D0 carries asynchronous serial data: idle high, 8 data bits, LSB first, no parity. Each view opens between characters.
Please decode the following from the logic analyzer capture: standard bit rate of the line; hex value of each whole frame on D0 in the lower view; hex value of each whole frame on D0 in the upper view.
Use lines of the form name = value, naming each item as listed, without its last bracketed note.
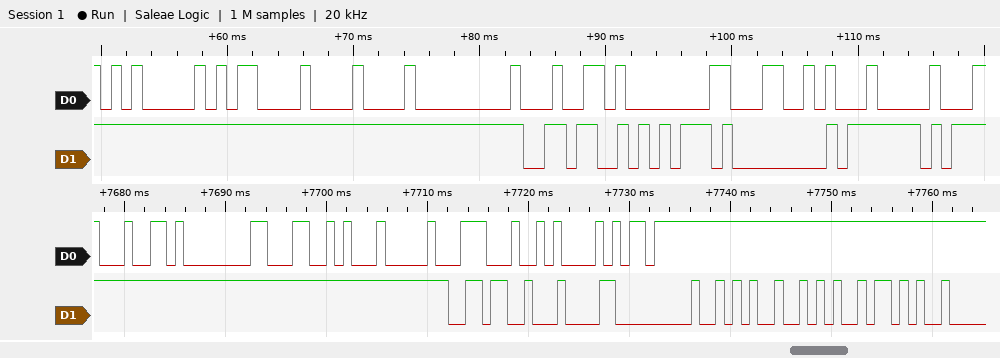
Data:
standard bit rate of the line = 1200 baud
hex value of each whole frame on D0 in the lower view = 64, 80, 4C, 04, 1C, 0A, ED
hex value of each whole frame on D0 in the upper view = 05, 0D, 08, 00, 64, 80, 4C, 04
